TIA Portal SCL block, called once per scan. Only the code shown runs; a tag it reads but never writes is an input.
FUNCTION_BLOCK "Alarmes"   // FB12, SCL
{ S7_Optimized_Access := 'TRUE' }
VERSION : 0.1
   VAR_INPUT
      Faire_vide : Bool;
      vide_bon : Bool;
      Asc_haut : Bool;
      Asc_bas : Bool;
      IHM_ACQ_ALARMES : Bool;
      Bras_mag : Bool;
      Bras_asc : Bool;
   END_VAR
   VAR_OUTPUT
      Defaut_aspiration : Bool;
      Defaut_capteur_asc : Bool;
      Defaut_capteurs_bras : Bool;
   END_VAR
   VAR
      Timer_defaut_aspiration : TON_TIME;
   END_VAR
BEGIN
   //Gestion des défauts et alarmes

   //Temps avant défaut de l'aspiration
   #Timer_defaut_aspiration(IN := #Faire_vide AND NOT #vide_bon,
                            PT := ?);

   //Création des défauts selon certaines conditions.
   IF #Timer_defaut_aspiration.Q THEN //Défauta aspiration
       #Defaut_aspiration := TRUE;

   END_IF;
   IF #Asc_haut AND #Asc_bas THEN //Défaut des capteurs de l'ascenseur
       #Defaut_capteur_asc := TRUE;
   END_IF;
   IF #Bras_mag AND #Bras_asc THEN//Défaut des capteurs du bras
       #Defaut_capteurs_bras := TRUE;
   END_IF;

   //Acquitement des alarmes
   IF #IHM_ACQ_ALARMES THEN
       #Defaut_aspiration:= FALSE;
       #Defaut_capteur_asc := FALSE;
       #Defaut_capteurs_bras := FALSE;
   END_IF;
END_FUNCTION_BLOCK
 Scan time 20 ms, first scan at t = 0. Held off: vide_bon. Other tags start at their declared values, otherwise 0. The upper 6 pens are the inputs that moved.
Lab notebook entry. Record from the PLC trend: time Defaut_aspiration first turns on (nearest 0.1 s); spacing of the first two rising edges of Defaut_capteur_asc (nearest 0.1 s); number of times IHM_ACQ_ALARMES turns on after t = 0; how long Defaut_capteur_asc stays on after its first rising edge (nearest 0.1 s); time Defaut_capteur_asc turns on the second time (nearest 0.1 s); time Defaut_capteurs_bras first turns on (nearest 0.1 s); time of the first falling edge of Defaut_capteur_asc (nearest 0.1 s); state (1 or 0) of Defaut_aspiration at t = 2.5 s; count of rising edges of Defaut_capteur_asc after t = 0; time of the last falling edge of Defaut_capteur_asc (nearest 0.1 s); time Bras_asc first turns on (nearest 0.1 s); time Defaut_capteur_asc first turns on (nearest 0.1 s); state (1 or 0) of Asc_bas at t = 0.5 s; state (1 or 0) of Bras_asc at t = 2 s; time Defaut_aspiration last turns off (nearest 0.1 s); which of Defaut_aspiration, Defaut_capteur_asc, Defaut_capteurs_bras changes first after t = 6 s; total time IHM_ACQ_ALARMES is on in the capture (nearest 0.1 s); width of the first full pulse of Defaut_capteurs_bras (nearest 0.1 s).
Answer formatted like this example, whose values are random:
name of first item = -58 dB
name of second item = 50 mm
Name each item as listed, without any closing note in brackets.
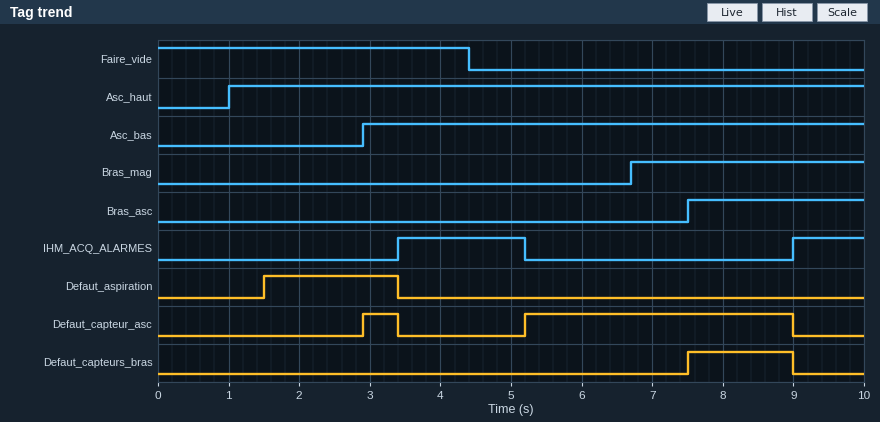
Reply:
time Defaut_aspiration first turns on = 1.5 s
spacing of the first two rising edges of Defaut_capteur_asc = 2.3 s
number of times IHM_ACQ_ALARMES turns on after t = 0 = 2
how long Defaut_capteur_asc stays on after its first rising edge = 0.5 s
time Defaut_capteur_asc turns on the second time = 5.2 s
time Defaut_capteurs_bras first turns on = 7.5 s
time of the first falling edge of Defaut_capteur_asc = 3.4 s
state (1 or 0) of Defaut_aspiration at t = 2.5 s = 1
count of rising edges of Defaut_capteur_asc after t = 0 = 2
time of the last falling edge of Defaut_capteur_asc = 9.0 s
time Bras_asc first turns on = 7.5 s
time Defaut_capteur_asc first turns on = 2.9 s
state (1 or 0) of Asc_bas at t = 0.5 s = 0
state (1 or 0) of Bras_asc at t = 2 s = 0
time Defaut_aspiration last turns off = 3.4 s
which of Defaut_aspiration, Defaut_capteur_asc, Defaut_capteurs_bras changes first after t = 6 s = Defaut_capteurs_bras
total time IHM_ACQ_ALARMES is on in the capture = 2.8 s
width of the first full pulse of Defaut_capteurs_bras = 1.5 s
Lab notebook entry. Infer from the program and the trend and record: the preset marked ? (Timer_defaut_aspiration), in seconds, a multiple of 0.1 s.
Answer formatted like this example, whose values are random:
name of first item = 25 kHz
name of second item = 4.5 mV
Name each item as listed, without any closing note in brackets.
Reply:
the preset marked ? (Timer_defaut_aspiration), in seconds, a multiple of 0.1 s = 1.5 s
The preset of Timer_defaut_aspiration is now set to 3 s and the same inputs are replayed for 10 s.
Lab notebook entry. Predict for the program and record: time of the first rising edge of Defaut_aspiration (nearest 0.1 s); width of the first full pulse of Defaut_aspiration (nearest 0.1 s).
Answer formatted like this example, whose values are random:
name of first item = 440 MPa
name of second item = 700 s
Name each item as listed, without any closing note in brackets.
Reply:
time of the first rising edge of Defaut_aspiration = 3.0 s
width of the first full pulse of Defaut_aspiration = 0.4 s
